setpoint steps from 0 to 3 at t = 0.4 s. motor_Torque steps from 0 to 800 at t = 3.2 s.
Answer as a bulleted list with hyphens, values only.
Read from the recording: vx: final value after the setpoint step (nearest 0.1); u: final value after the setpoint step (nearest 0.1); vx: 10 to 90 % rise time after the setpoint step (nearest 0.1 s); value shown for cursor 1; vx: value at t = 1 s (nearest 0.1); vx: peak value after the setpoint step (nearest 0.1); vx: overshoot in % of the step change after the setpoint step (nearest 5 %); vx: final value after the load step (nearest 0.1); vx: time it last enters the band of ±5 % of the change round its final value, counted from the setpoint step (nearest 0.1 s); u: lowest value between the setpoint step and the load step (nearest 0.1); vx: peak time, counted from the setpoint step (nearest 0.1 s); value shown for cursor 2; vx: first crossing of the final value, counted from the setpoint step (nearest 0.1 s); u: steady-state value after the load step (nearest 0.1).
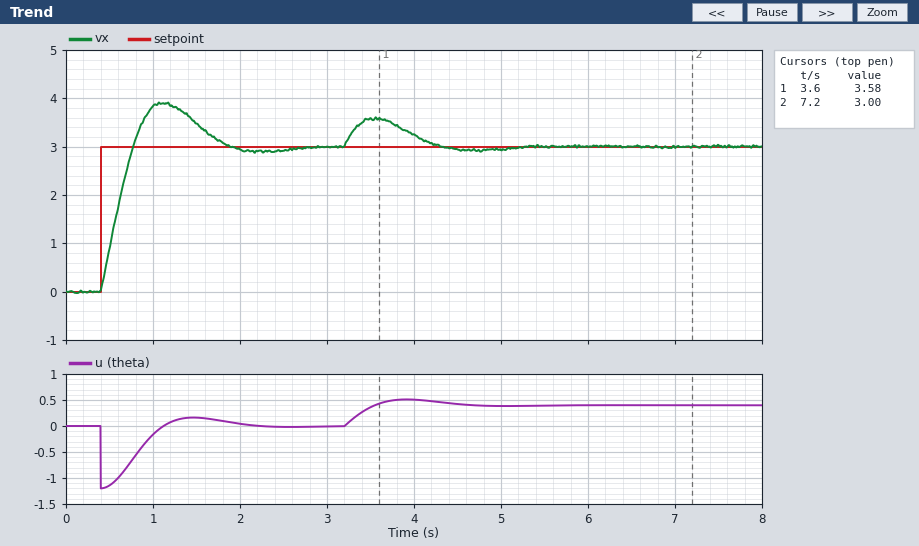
- 3.0
- 0.0
- 0.3 s
- 3.58
- 3.8
- 3.9
- 30 %
- 3.0
- 1.3 s
- -1.2
- 0.7 s
- 3.00
- 0.4 s
- 0.4
